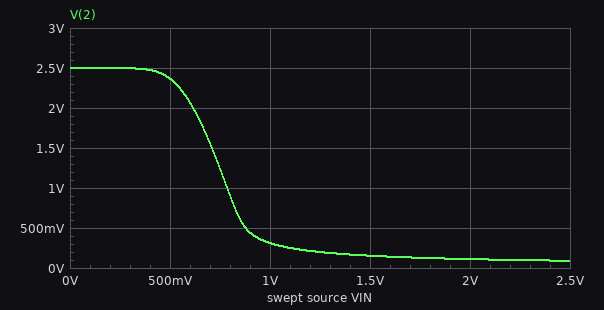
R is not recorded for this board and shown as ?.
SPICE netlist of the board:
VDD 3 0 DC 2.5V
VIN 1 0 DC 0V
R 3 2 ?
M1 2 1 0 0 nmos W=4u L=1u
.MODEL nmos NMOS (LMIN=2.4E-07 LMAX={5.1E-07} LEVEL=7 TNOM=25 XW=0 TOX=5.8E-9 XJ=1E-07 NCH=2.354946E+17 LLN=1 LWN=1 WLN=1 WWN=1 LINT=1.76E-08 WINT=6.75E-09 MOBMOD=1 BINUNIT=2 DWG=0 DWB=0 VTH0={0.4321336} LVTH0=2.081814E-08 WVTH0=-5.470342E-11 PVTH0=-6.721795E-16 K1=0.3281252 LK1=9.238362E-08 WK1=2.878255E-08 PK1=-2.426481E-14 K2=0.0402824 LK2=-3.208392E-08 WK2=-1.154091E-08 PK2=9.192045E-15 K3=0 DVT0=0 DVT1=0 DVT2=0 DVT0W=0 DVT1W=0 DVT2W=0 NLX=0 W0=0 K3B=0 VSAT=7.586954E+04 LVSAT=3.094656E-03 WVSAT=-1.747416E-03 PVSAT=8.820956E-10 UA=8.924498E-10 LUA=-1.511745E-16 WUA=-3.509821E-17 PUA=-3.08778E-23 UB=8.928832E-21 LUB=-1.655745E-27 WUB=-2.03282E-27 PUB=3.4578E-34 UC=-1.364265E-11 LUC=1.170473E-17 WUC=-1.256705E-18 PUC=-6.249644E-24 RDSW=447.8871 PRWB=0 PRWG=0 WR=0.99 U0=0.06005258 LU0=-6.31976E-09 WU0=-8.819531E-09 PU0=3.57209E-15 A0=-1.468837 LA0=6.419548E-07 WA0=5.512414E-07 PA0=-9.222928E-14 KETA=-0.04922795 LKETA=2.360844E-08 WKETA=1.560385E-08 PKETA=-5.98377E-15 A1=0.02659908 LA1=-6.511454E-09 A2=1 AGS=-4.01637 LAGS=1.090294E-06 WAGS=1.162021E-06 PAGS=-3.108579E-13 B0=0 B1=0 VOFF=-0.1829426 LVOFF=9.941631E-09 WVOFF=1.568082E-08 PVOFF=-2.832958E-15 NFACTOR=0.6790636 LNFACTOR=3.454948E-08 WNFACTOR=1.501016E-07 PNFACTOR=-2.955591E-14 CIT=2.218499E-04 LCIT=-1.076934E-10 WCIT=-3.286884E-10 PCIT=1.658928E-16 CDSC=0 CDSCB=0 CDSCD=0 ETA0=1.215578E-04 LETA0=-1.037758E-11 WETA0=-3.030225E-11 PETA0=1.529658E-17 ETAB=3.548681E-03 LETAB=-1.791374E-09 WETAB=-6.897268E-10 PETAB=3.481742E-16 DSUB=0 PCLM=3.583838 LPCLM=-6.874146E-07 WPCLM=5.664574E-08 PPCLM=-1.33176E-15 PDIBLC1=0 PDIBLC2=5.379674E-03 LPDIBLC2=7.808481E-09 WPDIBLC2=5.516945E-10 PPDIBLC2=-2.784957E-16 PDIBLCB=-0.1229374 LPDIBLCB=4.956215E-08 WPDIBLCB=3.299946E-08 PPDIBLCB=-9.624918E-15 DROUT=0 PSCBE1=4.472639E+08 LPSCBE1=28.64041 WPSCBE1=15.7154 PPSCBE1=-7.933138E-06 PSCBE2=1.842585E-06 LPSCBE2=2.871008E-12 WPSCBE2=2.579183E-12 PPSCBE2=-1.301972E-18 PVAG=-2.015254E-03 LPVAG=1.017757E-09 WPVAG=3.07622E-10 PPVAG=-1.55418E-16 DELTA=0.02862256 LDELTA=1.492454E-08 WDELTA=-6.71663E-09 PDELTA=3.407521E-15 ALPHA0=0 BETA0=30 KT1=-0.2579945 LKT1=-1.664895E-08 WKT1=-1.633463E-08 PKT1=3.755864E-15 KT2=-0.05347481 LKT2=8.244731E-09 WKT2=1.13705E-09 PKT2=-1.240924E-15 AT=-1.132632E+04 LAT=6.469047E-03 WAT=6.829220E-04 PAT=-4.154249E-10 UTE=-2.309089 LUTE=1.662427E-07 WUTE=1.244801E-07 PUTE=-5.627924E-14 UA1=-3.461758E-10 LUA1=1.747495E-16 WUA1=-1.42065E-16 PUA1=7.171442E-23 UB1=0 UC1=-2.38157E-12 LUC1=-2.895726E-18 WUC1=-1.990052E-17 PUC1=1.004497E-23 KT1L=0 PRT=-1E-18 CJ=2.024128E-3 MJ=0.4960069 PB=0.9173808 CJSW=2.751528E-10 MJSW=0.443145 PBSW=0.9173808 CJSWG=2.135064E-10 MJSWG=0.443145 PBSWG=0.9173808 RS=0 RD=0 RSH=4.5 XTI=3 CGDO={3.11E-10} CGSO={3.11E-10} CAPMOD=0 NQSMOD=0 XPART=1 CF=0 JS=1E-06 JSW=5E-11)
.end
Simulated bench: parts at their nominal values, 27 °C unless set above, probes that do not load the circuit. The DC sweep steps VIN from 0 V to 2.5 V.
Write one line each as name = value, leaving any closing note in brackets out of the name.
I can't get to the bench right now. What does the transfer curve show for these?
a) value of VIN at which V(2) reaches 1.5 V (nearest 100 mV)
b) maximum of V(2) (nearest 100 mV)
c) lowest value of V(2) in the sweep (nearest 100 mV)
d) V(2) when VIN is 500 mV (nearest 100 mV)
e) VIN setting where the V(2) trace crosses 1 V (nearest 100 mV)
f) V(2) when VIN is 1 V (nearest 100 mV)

value of VIN at which V(2) reaches 1.5 V = 700 mV
maximum of V(2) = 2.5 V
lowest value of V(2) in the sweep = 100 mV
V(2) when VIN is 500 mV = 2.4 V
VIN setting where the V(2) trace crosses 1 V = 800 mV
V(2) when VIN is 1 V = 300 mV
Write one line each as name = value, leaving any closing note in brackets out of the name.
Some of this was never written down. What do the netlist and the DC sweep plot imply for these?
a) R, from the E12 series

R, from the E12 series = 18 kΩ
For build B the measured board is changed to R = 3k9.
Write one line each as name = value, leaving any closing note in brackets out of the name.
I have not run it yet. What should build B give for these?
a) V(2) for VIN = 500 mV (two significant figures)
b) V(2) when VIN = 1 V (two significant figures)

V(2) for VIN = 500 mV = 2.5 V
V(2) when VIN = 1 V = 1.7 V
